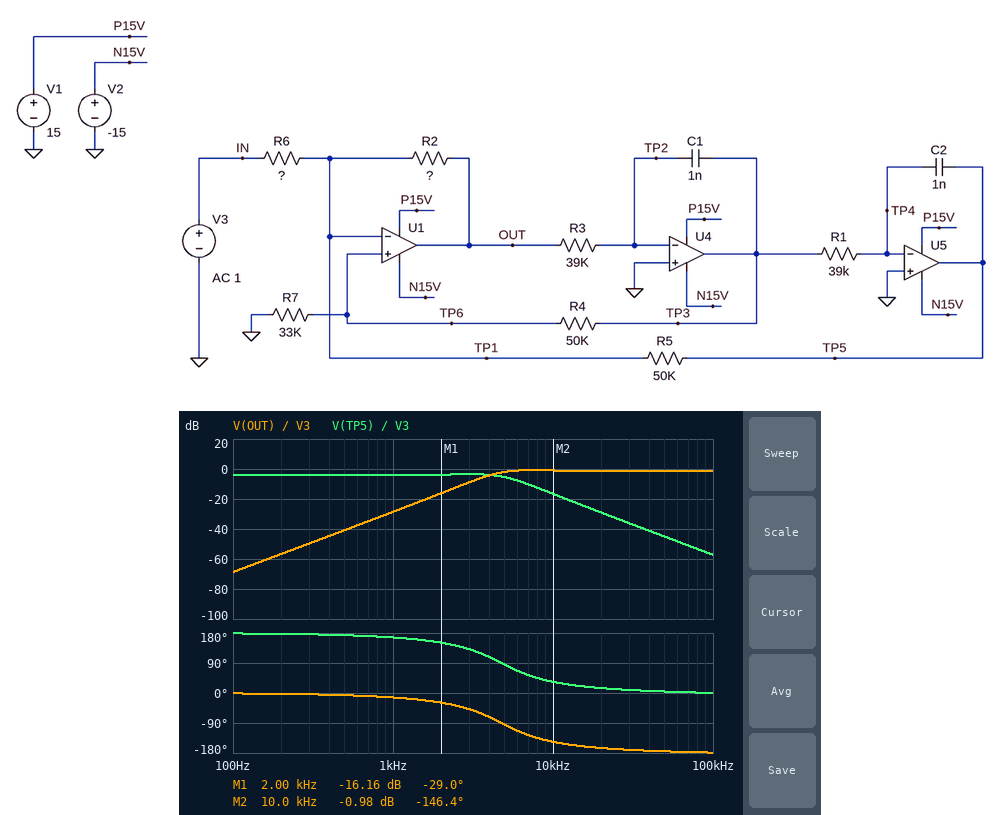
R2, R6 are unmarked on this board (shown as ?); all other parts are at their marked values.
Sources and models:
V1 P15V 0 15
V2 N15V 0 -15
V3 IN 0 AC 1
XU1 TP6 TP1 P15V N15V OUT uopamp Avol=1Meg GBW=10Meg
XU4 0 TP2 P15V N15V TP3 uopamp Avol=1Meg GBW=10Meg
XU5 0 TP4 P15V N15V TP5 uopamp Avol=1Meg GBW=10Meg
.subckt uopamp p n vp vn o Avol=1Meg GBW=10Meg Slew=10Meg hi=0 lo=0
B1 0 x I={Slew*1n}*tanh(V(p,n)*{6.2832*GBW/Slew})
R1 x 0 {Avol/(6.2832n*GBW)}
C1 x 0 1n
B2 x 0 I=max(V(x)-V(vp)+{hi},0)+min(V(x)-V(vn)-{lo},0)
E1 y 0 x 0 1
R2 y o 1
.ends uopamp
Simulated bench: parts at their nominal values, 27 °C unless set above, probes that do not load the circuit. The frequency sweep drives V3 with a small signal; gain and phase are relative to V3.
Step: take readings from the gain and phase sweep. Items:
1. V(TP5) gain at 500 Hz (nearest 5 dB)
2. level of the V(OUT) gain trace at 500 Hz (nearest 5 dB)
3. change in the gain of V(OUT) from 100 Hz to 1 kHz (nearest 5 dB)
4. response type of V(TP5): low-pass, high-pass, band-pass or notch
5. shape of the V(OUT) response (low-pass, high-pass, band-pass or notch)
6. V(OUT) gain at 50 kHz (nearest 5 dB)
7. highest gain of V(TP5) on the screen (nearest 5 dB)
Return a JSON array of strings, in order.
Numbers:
["-5 dB", "-40 dB", "40 dB", "low-pass", "high-pass", "0 dB", "-5 dB"]
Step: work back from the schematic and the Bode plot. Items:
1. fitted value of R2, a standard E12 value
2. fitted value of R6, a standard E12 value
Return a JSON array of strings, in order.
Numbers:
["68 kΩ", "82 kΩ"]
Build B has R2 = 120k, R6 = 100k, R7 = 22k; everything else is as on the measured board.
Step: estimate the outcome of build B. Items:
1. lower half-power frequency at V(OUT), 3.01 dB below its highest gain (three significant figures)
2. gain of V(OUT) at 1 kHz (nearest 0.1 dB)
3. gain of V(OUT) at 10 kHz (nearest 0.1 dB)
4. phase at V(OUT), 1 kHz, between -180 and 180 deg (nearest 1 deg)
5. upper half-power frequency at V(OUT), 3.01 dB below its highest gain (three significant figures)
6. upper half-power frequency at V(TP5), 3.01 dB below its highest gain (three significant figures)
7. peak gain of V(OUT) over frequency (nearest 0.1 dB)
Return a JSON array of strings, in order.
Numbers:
["5.35 kHz", "-30.3 dB", "3.2 dB", "-8 deg", "1.19 MHz", "7.48 kHz", "3.5 dB"]
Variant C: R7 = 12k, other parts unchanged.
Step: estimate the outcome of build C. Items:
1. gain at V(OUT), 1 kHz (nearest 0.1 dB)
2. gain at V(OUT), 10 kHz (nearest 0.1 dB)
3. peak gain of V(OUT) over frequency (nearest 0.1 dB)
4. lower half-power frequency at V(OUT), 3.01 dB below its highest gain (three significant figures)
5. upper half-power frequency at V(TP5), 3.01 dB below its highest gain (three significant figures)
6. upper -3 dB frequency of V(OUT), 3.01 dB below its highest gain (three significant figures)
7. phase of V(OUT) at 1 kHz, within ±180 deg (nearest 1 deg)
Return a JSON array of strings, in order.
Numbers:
["-28.4 dB", "0.2 dB", "4.3 dB", "4.07 kHz", "5.57 kHz", "8.02 kHz", "-7 deg"]
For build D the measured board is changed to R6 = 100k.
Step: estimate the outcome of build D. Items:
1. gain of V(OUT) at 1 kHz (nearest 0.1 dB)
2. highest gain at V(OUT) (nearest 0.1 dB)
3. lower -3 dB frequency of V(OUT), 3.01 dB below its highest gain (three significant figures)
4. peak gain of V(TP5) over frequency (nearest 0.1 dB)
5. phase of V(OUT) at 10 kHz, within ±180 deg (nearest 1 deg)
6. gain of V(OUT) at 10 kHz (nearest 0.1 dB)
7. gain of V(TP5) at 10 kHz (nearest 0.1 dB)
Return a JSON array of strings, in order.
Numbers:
["-30.3 dB", "-2.3 dB", "4.10 kHz", "-5.0 dB", "-148 deg", "-2.6 dB", "-18.2 dB"]
